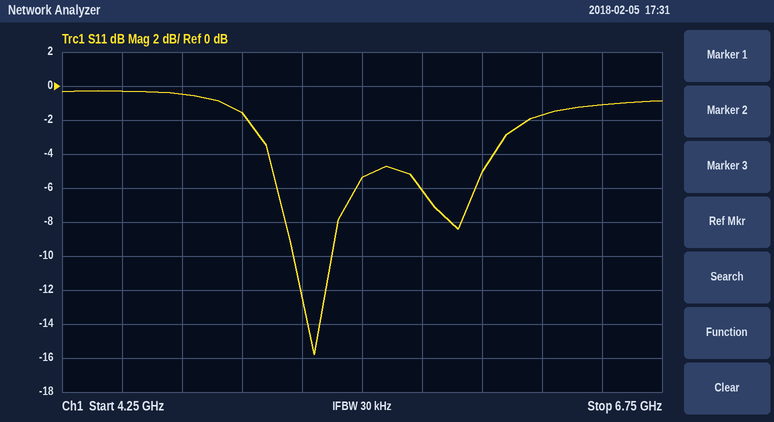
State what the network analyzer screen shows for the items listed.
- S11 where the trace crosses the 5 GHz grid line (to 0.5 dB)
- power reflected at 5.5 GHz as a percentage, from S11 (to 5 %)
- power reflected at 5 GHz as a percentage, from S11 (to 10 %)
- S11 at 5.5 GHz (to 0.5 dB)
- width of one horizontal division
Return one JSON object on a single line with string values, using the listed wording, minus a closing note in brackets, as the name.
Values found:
{"S11 where the trace crosses the 5 GHz grid line": "-1.5 dB", "power reflected at 5.5 GHz as a percentage, from S11": "30 %", "power reflected at 5 GHz as a percentage, from S11": "70 %", "S11 at 5.5 GHz": "-5.5 dB", "width of one horizontal division": "250 MHz"}
